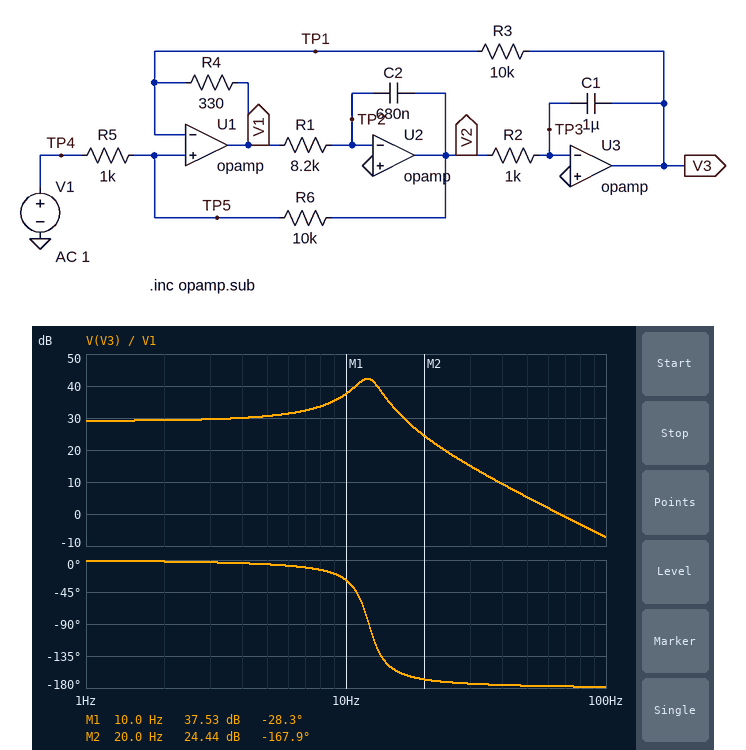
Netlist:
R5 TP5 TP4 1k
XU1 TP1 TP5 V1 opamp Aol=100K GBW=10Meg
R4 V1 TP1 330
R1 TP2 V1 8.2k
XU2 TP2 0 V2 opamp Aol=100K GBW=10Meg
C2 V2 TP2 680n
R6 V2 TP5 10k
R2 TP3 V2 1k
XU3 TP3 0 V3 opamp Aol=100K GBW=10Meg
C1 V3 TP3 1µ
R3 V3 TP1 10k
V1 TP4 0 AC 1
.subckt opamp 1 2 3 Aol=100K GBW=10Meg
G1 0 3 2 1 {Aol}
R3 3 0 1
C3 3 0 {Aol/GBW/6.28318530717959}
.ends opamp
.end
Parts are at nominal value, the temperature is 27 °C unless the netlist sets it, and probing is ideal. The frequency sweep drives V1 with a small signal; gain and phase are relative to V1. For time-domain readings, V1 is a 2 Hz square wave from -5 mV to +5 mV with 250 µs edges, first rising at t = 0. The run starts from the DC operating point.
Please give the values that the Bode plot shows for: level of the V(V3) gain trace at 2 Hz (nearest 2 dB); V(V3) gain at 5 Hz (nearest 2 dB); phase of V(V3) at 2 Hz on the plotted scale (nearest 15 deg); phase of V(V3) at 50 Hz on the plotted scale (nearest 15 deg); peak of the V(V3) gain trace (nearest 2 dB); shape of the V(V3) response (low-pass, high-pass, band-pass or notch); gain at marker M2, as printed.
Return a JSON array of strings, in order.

["30 dB", "30 dB", "0 deg", "-180 deg", "42 dB", "low-pass", "24.44 dB"]
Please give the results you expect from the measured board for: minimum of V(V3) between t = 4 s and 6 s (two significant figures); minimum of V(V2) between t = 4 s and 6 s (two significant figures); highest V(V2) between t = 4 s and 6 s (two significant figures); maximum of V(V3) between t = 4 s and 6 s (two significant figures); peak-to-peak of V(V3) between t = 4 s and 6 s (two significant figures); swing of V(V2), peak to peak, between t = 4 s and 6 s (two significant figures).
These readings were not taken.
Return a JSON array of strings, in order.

["-320 mV", "-17 mV", "17 mV", "320 mV", "640 mV", "33 mV"]
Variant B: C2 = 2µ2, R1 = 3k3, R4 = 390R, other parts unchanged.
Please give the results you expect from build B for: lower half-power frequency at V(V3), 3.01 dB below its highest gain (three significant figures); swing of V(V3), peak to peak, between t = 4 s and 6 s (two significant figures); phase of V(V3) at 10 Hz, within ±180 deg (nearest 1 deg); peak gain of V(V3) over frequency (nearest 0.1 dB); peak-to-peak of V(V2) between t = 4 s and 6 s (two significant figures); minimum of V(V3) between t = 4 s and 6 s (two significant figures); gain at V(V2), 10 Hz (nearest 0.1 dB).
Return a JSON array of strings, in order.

["10.5 Hz", "560 mV", "-30 deg", "42.7 dB", "27 mV", "-280 mV", "13.9 dB"]
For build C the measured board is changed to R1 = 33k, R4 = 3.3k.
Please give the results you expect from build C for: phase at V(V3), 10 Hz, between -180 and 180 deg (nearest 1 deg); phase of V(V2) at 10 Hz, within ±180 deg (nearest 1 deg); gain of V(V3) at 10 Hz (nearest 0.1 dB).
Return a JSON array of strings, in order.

["-2 deg", "-92 deg", "14.0 dB"]
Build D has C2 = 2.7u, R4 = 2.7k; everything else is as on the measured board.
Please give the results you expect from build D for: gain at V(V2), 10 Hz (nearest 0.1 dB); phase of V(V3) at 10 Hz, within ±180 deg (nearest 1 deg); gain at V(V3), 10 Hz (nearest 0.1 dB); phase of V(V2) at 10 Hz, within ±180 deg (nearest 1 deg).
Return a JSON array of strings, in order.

["-8.0 dB", "-2 deg", "16.0 dB", "-92 deg"]
